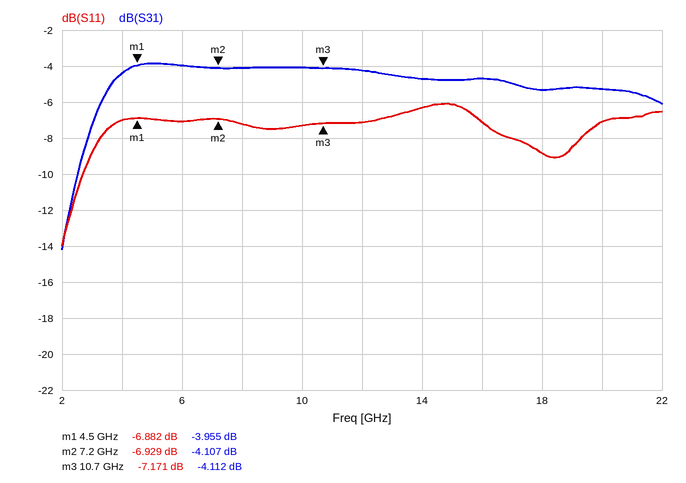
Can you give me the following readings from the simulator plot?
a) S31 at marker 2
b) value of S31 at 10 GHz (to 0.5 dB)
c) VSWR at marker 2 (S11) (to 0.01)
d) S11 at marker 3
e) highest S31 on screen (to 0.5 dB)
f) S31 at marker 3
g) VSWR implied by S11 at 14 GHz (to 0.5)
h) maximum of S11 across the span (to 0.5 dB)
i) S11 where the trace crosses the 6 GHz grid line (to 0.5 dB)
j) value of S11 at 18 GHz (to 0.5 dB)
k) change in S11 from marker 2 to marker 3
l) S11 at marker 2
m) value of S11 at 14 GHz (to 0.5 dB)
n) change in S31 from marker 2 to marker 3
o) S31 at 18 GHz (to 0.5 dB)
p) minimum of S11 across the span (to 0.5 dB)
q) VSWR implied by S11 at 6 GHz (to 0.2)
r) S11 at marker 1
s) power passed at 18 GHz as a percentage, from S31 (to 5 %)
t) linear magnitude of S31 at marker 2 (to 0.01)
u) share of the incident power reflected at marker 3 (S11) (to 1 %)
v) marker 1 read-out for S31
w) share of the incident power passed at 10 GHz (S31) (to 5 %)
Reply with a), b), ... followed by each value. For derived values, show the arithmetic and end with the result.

a) -4.107 dB
b) -4.0 dB
c) (1 + 0.4503)/(1 − 0.4503) ≈ 2.64
d) -7.171 dB
e) -4.0 dB
f) -4.112 dB
g) |Γ| = 10^(-6.5/20) = 0.4732; VSWR = (1 + 0.4732)/(1 − 0.4732) ≈ 2.80, so 3.0 to the nearest 0.5
h) -6.0 dB
i) -7.0 dB
j) -9.0 dB
k) -7.171 − (-6.929) = -0.242 dB
l) -6.929 dB
m) -6.5 dB
n) -4.112 − (-4.107) = -0.005 dB
o) -5.5 dB
p) -14.0 dB
q) |Γ| = 10^(-7/20) = 0.4467; VSWR = (1 + 0.4467)/(1 − 0.4467) ≈ 2.6
r) -6.882 dB
s) 10^(-5.5/10) ≈ 28.2 %, so 30 % to the nearest 5 %
t) 10^(-4.107/20) ≈ 0.62
u) 10^(-7.171/10) ≈ 19 %
v) -3.955 dB
w) 10^(-4/10) ≈ 40 %
